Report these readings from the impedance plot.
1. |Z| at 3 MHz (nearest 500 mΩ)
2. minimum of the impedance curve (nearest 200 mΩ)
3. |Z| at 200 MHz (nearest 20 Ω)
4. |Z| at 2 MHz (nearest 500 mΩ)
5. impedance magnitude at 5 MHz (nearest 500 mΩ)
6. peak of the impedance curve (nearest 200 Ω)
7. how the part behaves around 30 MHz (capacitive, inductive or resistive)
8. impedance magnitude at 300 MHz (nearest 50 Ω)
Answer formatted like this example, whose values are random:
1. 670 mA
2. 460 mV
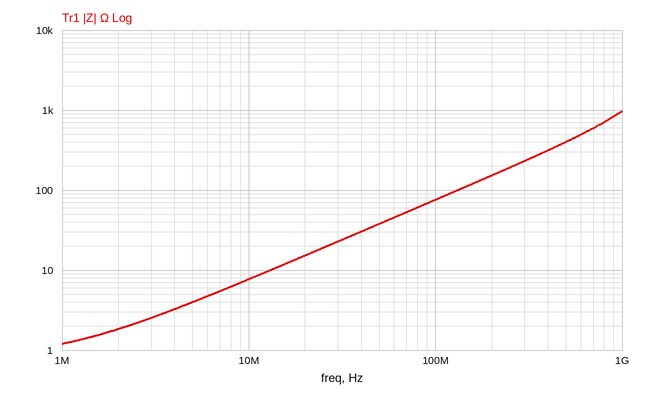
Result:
1. 2.5 Ω
2. 1.2 Ω
3. 160 Ω
4. 2.0 Ω
5. 4.0 Ω
6. 1.0 kΩ
7. inductive
8. 250 Ω
